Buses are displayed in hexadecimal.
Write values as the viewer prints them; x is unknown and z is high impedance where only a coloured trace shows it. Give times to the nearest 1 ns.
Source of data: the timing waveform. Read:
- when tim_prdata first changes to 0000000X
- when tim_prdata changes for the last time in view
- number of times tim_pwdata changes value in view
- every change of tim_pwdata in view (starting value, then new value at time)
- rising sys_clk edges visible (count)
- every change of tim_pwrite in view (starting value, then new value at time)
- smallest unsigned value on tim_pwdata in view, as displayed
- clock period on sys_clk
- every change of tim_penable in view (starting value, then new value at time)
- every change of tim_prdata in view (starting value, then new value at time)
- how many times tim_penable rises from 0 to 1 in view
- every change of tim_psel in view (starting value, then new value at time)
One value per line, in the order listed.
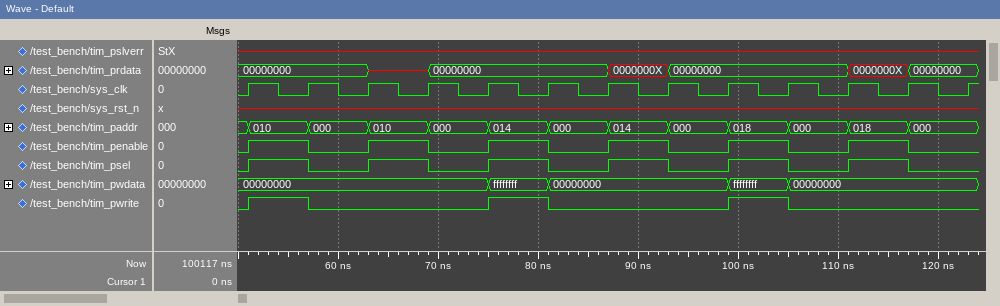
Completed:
87 ns
117 ns
4
00000000, ffffffff at 75 ns, 00000000 at 81 ns, ffffffff at 99 ns, 00000000 at 105 ns
13
0, 1 at 51 ns, 0 at 57 ns, 1 at 75 ns, 0 at 81 ns, 1 at 99 ns, 0 at 105 ns
00000000
6 ns
0, 1 at 51 ns, 0 at 57 ns, 1 at 63 ns, 0 at 69 ns, 1 at 75 ns, 0 at 81 ns, 1 at 87 ns, 0 at 93 ns, 1 at 99 ns, 0 at 105 ns, 1 at 111 ns, 0 at 117 ns
00000000, x at 63 ns, 00000000 at 69 ns, 0000000X at 87 ns, 00000000 at 93 ns, 0000000X at 111 ns, 00000000 at 117 ns
6
0, 1 at 51 ns, 0 at 57 ns, 1 at 63 ns, 0 at 69 ns, 1 at 75 ns, 0 at 81 ns, 1 at 87 ns, 0 at 93 ns, 1 at 99 ns, 0 at 105 ns, 1 at 111 ns, 0 at 117 ns
